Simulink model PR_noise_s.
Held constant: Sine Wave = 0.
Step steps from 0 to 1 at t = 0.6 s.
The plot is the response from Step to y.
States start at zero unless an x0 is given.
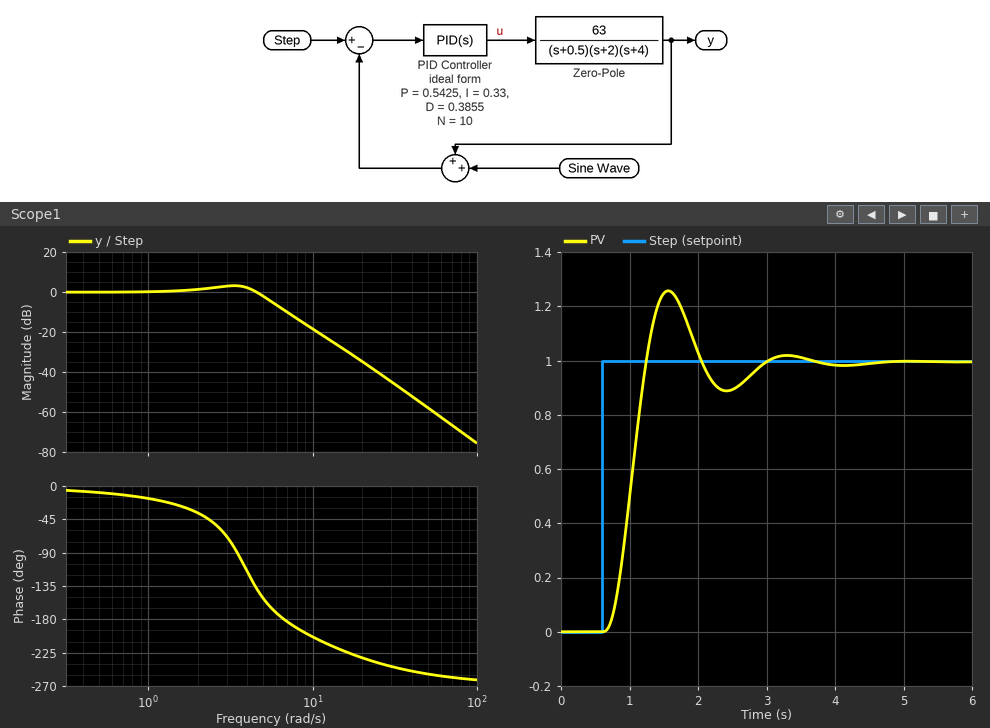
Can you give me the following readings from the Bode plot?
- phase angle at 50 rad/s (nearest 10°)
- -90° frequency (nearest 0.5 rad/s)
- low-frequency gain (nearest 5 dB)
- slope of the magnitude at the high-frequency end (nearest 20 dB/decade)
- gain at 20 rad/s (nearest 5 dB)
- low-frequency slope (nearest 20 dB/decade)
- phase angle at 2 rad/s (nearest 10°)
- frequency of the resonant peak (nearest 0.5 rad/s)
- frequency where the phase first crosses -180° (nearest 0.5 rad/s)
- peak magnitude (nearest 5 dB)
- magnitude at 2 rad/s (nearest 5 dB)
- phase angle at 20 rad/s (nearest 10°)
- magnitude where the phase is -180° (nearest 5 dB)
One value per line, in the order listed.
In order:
-250°
3.5 rad/s
0 dB
-60 dB/decade
-35 dB
0 dB/decade
-40°
3.5 rad/s
6.5 rad/s
5 dB
0 dB
-230°
-10 dB
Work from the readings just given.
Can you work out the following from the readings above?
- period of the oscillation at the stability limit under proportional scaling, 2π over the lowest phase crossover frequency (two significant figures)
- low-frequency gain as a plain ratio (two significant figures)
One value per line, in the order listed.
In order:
0.97 s
1.0
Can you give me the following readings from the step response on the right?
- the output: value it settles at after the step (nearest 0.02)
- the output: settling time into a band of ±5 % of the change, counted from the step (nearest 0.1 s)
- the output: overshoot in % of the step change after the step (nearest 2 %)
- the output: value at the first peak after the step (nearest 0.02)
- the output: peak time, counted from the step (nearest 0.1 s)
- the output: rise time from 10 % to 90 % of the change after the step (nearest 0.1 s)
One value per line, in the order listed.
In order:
1.00
2.2 s
26 %
1.26
1.0 s
0.4 s
